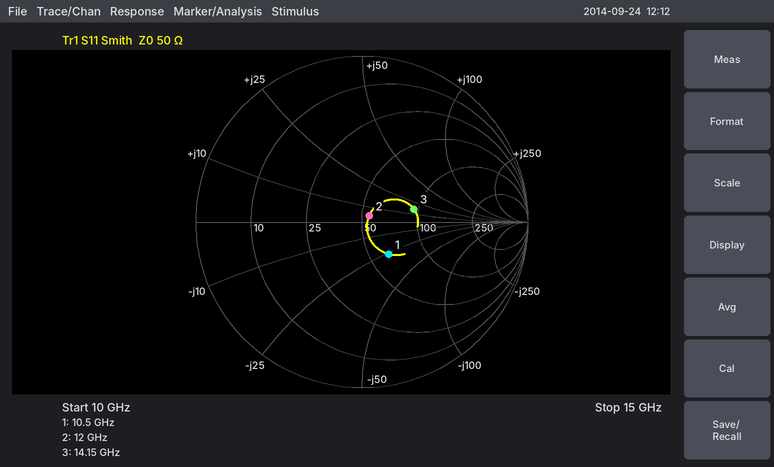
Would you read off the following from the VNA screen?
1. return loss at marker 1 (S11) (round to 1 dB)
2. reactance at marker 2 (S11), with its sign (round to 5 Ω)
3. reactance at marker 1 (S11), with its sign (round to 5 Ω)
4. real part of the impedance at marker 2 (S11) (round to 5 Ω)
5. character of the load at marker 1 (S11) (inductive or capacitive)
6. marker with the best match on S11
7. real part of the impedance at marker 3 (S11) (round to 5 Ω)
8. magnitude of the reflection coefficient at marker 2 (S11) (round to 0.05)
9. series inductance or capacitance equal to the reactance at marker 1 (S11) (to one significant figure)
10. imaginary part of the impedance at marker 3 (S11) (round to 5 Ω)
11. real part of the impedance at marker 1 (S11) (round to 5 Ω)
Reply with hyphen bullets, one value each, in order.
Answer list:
- 12 dB
- +5 Ω
- -25 Ω
- 55 Ω
- capacitive
- marker 2
- 95 Ω
- 0.05
- 600 fF
- +15 Ω
- 65 Ω
